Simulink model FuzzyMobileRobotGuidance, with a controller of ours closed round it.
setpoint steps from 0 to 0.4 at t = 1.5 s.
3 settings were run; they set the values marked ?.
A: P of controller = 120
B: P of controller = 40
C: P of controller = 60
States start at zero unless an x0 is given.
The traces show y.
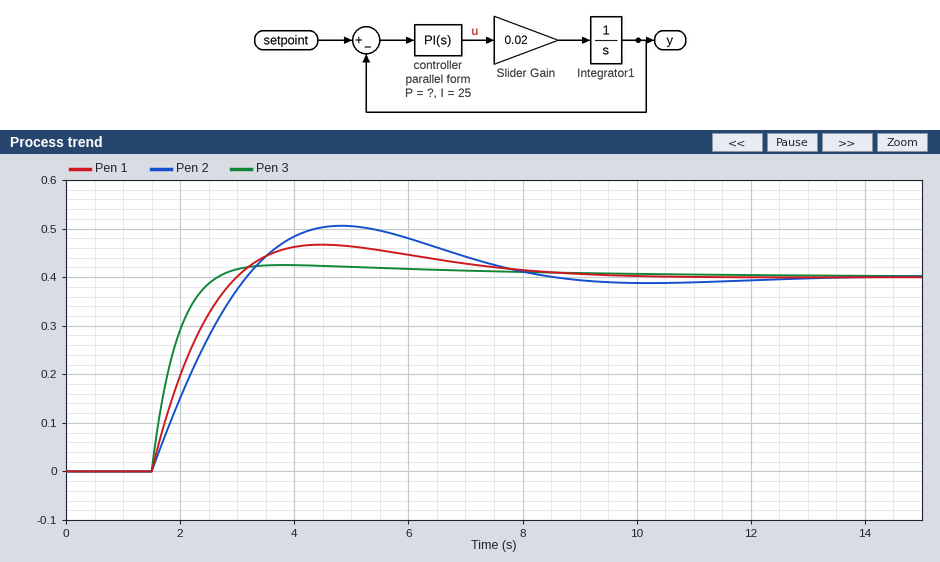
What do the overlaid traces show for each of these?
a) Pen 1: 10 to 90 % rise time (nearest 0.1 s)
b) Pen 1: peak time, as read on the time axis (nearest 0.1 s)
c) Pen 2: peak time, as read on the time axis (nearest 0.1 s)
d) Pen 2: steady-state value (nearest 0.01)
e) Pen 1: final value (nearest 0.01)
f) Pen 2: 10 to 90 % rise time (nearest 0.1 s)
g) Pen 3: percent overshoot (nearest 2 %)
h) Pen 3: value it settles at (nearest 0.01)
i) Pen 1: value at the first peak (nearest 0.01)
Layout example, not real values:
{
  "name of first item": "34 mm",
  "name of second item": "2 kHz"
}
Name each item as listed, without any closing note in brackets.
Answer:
{
  "Pen 1: 10 to 90 % rise time": "1.1 s",
  "Pen 1: peak time, as read on the time axis": "4.5 s",
  "Pen 2: peak time, as read on the time axis": "4.8 s",
  "Pen 2: steady-state value": "0.40",
  "Pen 1: final value": "0.40",
  "Pen 2: 10 to 90 % rise time": "1.3 s",
  "Pen 3: percent overshoot": "6 %",
  "Pen 3: value it settles at": "0.40",
  "Pen 1: value at the first peak": "0.47"
}
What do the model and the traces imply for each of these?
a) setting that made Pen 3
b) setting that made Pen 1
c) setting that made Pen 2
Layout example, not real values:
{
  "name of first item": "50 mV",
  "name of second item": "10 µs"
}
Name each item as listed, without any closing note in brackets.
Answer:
{
  "setting that made Pen 3": "A",
  "setting that made Pen 1": "C",
  "setting that made Pen 2": "B"
}
